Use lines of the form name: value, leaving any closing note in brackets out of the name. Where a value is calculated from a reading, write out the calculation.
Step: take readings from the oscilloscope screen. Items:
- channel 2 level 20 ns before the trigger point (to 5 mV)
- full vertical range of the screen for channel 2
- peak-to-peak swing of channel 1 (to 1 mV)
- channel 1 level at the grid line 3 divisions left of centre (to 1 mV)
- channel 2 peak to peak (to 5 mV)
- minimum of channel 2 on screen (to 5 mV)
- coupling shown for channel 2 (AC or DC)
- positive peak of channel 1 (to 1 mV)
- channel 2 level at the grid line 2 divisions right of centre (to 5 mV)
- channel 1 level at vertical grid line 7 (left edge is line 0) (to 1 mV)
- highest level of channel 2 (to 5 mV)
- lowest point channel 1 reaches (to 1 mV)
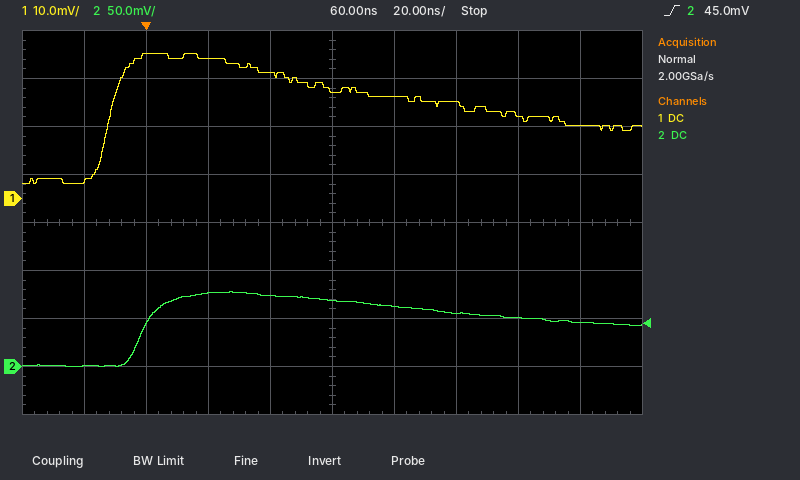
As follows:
channel 2 level 20 ns before the trigger point: 0 mV
full vertical range of the screen for channel 2: 400 mV
peak-to-peak swing of channel 1: 30 mV − (3 mV) = 27 mV
channel 1 level at the grid line 3 divisions left of centre: 30 mV
channel 2 peak to peak: 80 mV − (0 mV) = 80 mV
minimum of channel 2 on screen: 0 mV
coupling shown for channel 2: DC
positive peak of channel 1: 30 mV
channel 2 level at the grid line 2 divisions right of centre: 55 mV
channel 1 level at vertical grid line 7 (left edge is line 0): 20 mV
highest level of channel 2: 80 mV
lowest point channel 1 reaches: 3 mV
